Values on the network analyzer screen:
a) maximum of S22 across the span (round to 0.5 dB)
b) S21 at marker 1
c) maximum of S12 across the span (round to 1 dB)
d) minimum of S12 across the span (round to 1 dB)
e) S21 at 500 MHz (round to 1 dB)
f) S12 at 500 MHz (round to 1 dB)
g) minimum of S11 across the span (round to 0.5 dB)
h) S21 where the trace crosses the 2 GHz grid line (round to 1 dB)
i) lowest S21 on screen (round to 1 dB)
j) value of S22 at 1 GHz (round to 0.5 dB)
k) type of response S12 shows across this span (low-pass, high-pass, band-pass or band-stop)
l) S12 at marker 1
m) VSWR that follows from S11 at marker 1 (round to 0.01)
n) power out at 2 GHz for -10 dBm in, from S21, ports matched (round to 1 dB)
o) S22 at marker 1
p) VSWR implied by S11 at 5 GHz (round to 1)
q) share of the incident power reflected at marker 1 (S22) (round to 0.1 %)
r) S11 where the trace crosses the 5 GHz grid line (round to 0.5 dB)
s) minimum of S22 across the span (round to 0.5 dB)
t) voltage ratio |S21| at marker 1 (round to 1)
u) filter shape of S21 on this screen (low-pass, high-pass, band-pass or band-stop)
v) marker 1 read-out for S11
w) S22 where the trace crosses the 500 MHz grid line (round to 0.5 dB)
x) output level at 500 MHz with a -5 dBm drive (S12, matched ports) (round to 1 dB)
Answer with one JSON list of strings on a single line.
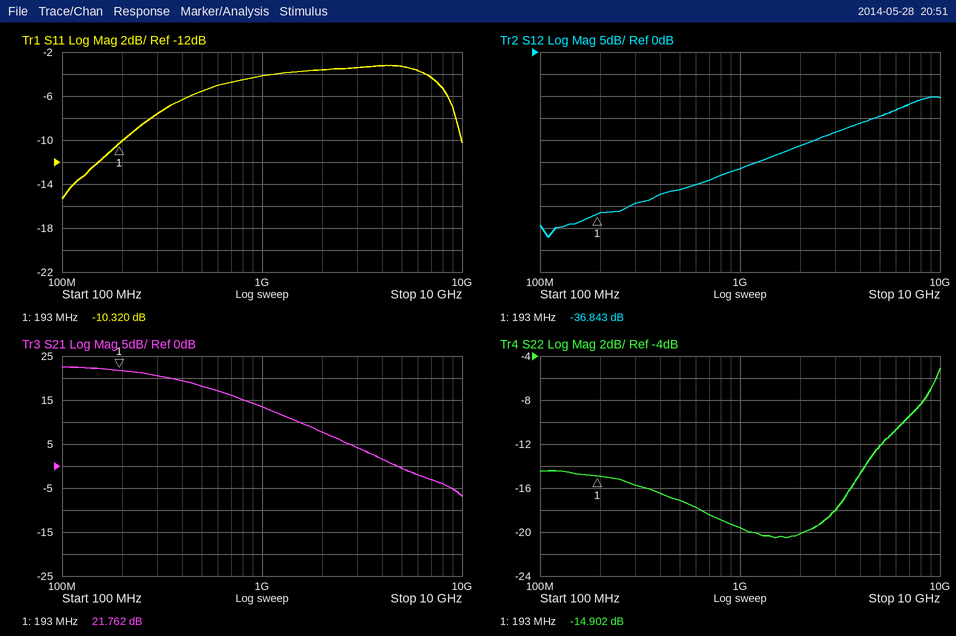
["-5.0 dB", "21.762 dB", "-10 dB", "-42 dB", "18 dB", "-31 dB", "-15.5 dB", "8 dB", "-7 dB", "-19.5 dB", "high-pass", "-36.843 dB", "1.88", "-2 dBm", "-14.902 dB", "5", "3.2 %", "-3.5 dB", "-20.5 dB", "12", "low-pass", "-10.320 dB", "-17.0 dB", "-36 dBm"]
